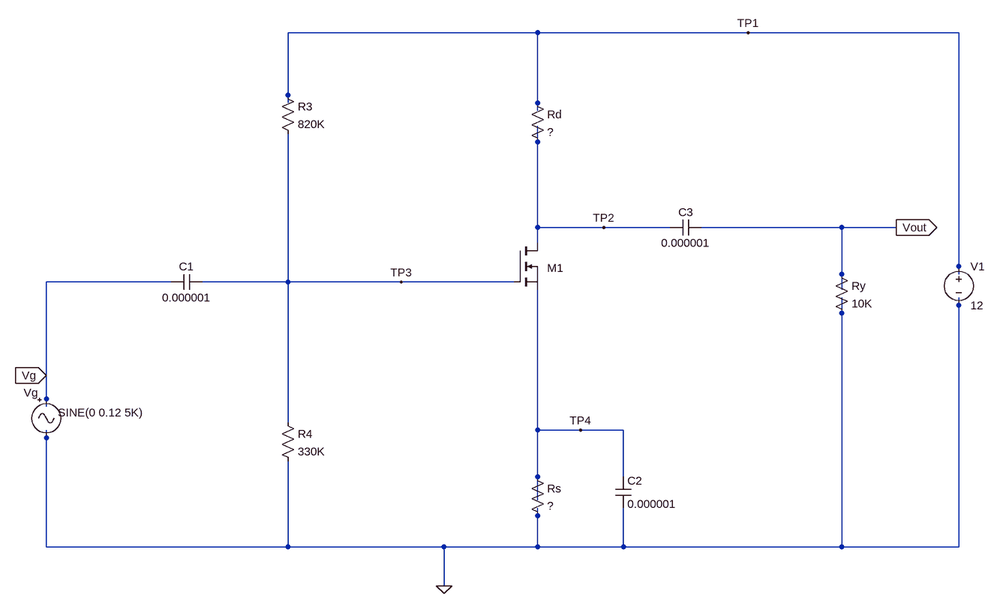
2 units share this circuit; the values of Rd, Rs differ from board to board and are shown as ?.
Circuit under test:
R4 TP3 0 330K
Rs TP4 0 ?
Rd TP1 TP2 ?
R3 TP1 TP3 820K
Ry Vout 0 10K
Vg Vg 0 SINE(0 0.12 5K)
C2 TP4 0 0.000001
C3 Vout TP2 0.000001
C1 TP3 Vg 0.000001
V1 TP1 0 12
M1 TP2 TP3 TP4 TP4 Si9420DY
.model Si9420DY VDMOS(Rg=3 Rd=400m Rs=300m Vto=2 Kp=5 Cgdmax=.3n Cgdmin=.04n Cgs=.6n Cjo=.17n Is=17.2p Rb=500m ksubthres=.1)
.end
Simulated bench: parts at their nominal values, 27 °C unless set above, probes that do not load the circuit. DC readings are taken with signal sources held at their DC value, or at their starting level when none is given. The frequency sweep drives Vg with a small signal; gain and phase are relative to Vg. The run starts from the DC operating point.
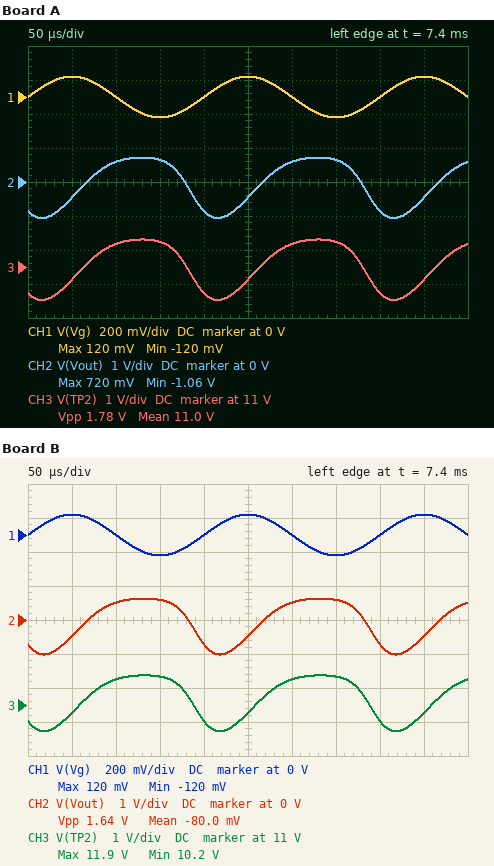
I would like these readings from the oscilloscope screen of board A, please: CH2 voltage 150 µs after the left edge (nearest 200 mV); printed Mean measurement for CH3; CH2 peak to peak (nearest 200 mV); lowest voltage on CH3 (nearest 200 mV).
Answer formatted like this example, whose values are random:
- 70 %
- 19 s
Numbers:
- 600 mV
- 11.0 V
- 1.8 V
- 10.0 V
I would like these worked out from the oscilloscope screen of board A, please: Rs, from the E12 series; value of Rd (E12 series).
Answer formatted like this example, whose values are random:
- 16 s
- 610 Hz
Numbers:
- 560 Ω
- 330 Ω
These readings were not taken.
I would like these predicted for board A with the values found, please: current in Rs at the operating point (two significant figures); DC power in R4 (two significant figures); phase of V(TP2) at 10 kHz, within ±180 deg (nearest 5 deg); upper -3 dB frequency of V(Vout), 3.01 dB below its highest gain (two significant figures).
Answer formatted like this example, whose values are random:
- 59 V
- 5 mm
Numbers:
- 2.7 mA
- 36 µW
- -145 deg
- 4.6 MHz
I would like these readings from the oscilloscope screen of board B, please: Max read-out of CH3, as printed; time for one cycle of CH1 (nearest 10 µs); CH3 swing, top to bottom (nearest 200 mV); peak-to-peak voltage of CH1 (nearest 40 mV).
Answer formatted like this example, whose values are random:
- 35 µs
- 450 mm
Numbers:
- 11.9 V
- 200 µs
- 1.6 V
- 240 mV
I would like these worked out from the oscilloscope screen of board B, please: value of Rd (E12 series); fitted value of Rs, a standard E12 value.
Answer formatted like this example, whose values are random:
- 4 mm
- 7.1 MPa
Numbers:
- 330 Ω
- 680 Ω
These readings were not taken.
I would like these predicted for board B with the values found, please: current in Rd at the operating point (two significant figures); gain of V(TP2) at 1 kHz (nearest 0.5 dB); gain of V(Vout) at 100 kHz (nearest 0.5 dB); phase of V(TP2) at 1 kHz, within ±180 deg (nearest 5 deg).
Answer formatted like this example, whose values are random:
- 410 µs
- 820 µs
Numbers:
- 2.3 mA
- 6.0 dB
- 22.0 dB
- -110 deg
